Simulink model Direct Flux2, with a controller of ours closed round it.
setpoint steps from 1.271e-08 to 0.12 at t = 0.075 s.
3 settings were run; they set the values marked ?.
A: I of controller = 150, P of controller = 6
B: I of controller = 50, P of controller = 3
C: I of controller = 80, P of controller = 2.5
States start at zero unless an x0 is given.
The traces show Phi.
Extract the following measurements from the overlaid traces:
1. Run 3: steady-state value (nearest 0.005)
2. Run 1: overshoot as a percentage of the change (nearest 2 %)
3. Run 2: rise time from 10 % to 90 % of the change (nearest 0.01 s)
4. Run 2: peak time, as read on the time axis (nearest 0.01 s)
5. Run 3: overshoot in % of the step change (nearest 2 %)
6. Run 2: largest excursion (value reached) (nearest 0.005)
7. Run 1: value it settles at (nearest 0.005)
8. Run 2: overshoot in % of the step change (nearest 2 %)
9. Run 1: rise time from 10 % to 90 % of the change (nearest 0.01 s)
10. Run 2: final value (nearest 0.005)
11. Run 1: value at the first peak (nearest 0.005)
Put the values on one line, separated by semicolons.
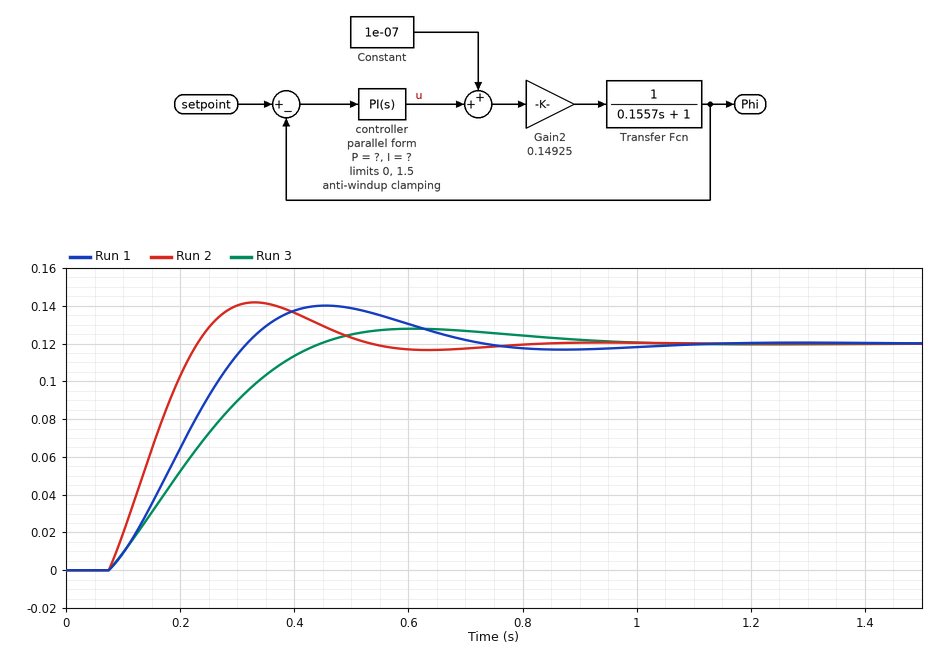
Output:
0.120; 16 %; 0.12 s; 0.33 s; 6 %; 0.140; 0.120; 18 %; 0.18 s; 0.120; 0.140
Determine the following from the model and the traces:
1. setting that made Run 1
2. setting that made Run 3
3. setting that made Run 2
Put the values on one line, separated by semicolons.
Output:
C; B; A
